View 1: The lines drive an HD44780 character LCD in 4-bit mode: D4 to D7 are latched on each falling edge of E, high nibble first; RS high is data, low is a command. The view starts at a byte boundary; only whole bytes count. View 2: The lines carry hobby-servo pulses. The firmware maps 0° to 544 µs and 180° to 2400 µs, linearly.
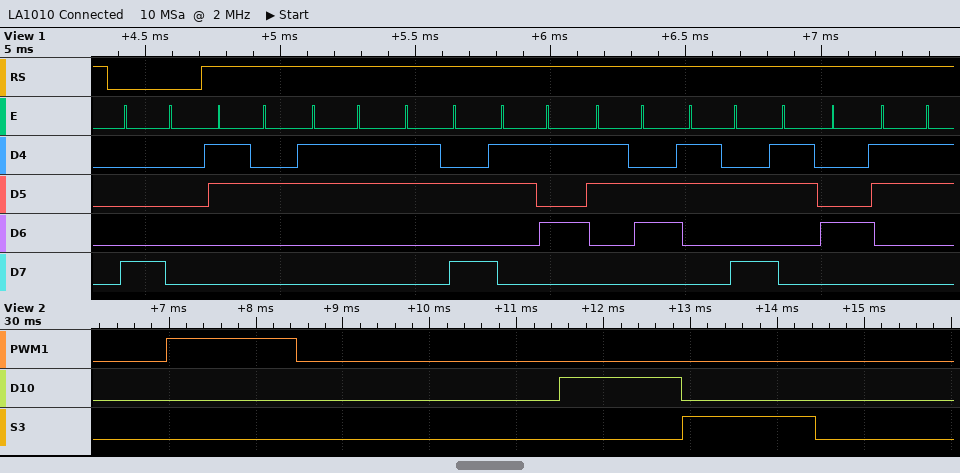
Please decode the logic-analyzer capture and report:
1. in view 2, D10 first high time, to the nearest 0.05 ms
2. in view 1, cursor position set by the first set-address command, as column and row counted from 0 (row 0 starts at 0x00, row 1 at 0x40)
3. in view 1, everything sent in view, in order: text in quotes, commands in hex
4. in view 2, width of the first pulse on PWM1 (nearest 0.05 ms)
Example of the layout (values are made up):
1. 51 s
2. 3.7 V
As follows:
1. 1.40 ms
2. column 0, row 0
3. 0x80 "23:56:43"
4. 1.50 ms
